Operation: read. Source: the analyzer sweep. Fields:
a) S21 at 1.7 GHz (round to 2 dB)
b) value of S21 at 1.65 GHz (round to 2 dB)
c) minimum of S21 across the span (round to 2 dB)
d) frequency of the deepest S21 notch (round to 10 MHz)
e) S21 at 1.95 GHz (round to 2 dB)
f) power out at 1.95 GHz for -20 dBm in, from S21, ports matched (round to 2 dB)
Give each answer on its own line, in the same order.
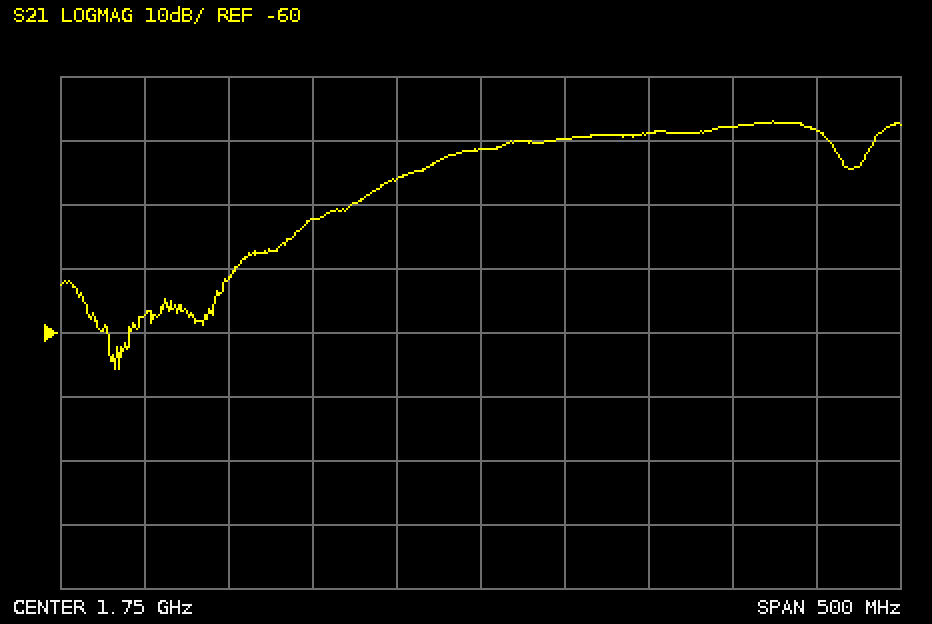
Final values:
-36 dB
-42 dB
-66 dB
1.53 GHz
-28 dB
-48 dBm
